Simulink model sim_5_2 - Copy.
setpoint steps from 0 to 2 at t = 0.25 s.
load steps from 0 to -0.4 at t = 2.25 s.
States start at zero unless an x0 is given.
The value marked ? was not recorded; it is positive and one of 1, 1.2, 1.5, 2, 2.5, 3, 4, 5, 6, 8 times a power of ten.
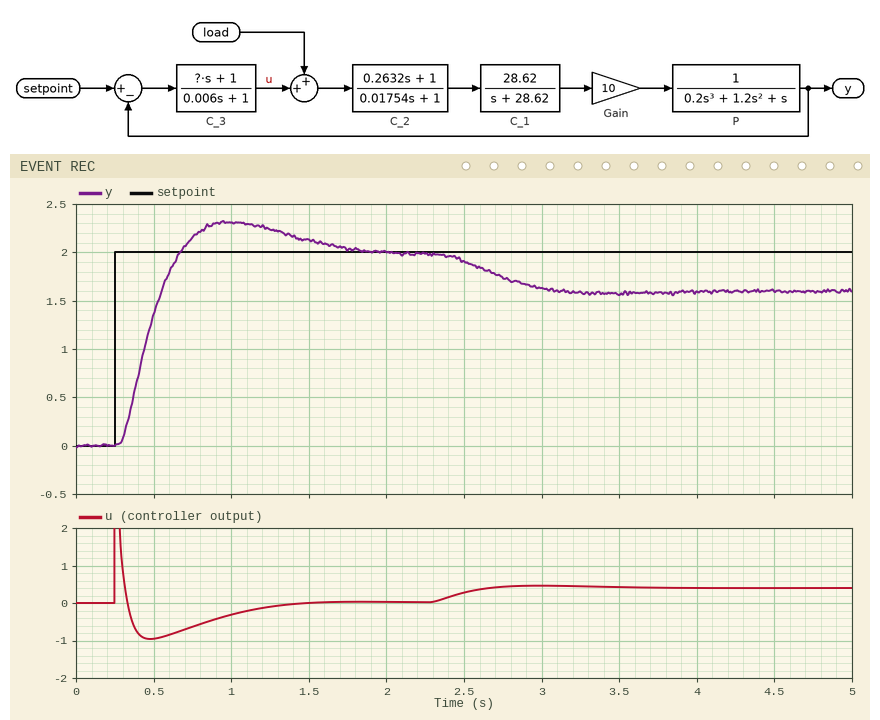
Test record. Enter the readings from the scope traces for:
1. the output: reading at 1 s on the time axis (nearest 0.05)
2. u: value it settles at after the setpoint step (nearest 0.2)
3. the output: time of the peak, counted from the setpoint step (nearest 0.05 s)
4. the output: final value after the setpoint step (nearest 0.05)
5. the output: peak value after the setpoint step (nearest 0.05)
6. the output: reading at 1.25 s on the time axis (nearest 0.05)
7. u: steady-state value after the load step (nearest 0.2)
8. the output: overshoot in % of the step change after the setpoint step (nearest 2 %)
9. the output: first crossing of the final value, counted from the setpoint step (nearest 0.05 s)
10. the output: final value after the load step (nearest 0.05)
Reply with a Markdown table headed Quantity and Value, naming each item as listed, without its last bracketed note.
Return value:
| Quantity | Value |
|---|---|
| the output: reading at 1 s on the time axis | 2.30 |
| u: value it settles at after the setpoint step | 0.0 |
| the output: time of the peak, counted from the setpoint step | 0.75 s |
| the output: final value after the setpoint step | 2.00 |
| the output: peak value after the setpoint step | 2.30 |
| the output: reading at 1.25 s on the time axis | 2.25 |
| u: steady-state value after the load step | 0.4 |
| the output: overshoot in % of the step change after the setpoint step | 16 % |
| the output: first crossing of the final value, counted from the setpoint step | 0.40 s |
| the output: final value after the load step | 1.60 |
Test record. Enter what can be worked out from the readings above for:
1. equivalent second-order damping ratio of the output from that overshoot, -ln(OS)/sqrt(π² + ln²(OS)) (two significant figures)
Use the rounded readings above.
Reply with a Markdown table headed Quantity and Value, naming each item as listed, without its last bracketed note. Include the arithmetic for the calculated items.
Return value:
| Quantity | Value |
|---|---|
| equivalent second-order damping ratio of the output from that overshoot, -ln(OS)/sqrt(π² + ln²(OS)) | ln(0.16) = -1.833; 1.833 / sqrt(9.870 + 3.358) = 0.50 |
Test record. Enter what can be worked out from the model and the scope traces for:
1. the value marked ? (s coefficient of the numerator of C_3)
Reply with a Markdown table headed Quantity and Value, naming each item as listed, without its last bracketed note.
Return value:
| Quantity | Value |
|---|---|
| the value marked ? | 0.3 |
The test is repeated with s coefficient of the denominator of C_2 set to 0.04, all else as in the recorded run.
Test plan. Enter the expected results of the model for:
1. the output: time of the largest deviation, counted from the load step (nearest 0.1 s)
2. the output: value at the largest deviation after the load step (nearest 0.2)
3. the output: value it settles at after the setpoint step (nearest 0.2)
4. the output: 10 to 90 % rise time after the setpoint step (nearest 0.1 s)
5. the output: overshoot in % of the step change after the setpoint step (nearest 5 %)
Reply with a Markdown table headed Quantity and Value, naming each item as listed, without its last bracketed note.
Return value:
| Quantity | Value |
|---|---|
| the output: time of the largest deviation, counted from the load step | 1.2 s |
| the output: value at the largest deviation after the load step | 1.6 |
| the output: value it settles at after the setpoint step | 2.0 |
| the output: 10 to 90 % rise time after the setpoint step | 0.3 s |
| the output: overshoot in % of the step change after the setpoint step | 20 % |
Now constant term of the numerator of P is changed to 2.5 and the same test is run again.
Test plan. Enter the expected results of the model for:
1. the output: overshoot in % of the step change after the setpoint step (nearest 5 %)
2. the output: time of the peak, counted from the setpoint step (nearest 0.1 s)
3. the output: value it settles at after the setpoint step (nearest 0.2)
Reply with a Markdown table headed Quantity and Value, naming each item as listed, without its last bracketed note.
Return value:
| Quantity | Value |
|---|---|
| the output: overshoot in % of the step change after the setpoint step | 20 % |
| the output: time of the peak, counted from the setpoint step | 0.3 s |
| the output: value it settles at after the setpoint step | 2.0 |
